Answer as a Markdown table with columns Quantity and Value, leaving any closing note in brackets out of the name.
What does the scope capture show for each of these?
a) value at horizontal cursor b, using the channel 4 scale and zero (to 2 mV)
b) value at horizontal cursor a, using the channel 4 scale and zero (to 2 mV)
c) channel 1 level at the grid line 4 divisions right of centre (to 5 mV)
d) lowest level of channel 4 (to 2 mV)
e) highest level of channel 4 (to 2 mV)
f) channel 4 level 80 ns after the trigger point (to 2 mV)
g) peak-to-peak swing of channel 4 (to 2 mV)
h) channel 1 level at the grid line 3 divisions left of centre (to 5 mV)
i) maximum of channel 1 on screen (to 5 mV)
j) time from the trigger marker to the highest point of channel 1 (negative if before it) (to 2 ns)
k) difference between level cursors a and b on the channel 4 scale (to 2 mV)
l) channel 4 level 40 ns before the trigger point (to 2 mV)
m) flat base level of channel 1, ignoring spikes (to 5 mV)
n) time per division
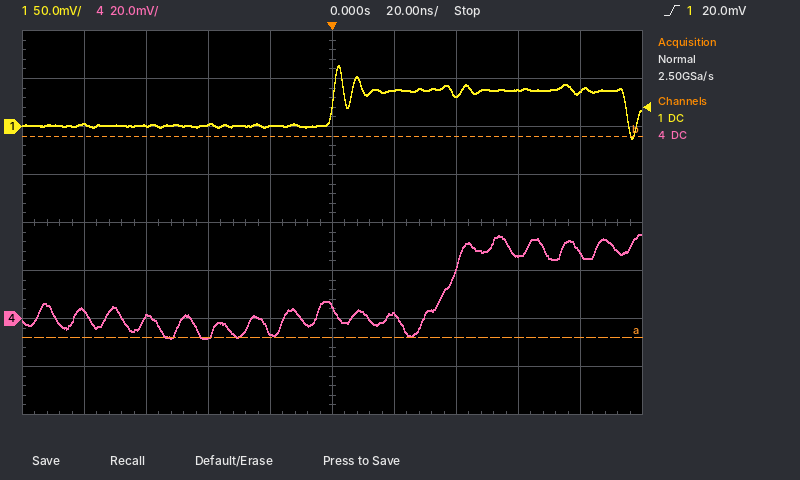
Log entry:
| Quantity | Value |
|---|---|
| value at horizontal cursor b, using the channel 4 scale and zero | 76 mV |
| value at horizontal cursor a, using the channel 4 scale and zero | -8 mV |
| channel 1 level at the grid line 4 divisions right of centre | 35 mV |
| lowest level of channel 4 | -8 mV |
| highest level of channel 4 | 36 mV |
| channel 4 level 80 ns after the trigger point | 28 mV |
| peak-to-peak swing of channel 4 | 44 mV |
| channel 1 level at the grid line 3 divisions left of centre | 0 mV |
| maximum of channel 1 on screen | 65 mV |
| time from the trigger marker to the highest point of channel 1 (negative if before it) | +2 ns |
| difference between level cursors a and b on the channel 4 scale | 84 mV |
| channel 4 level 40 ns before the trigger point | -8 mV |
| flat base level of channel 1, ignoring spikes | 0 mV |
| time per division | 20 ns |
